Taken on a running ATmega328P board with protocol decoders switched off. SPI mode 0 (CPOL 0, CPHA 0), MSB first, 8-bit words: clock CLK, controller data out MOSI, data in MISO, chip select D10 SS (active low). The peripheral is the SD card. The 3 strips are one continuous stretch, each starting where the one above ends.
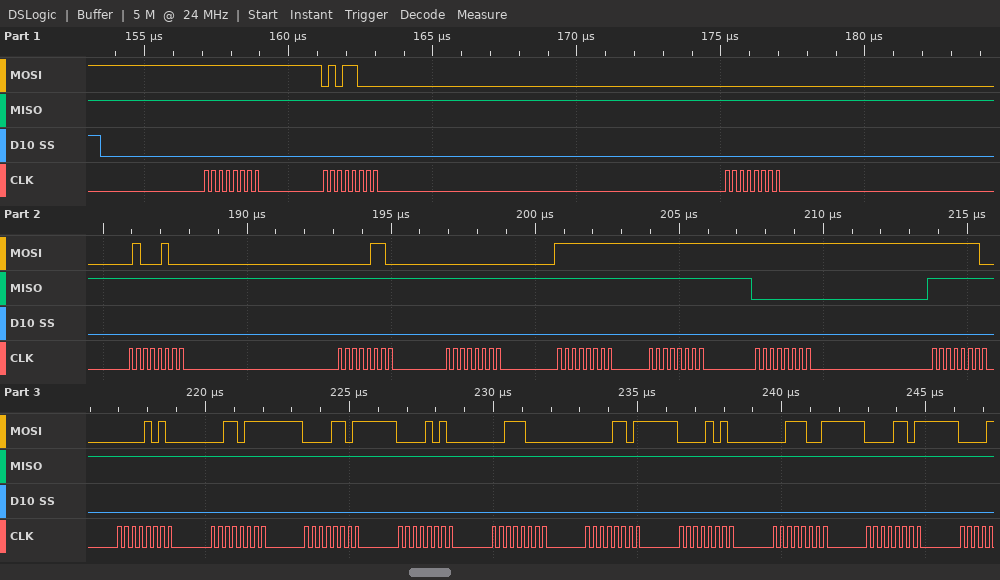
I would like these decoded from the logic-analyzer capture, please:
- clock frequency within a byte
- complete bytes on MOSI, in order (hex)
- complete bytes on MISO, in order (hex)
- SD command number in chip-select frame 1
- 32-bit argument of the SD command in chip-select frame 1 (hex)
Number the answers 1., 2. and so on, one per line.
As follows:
1. 4 MHz
2. 0xFF 0x58 0x00 0x44 0x06 0x00 0xFF 0xFF 0xFF 0xFE 0x0A 0x37 0x0D 0x0A 0x38 0x0D 0x0A 0x39 0x0D
3. 0xFF 0xFF 0xFF 0xFF 0xFF 0xFF 0xFF 0xFF 0x00 0xFF 0xFF 0xFF 0xFF 0xFF 0xFF 0xFF 0xFF 0xFF 0xFF
4. CMD24
5. 0x00440600
